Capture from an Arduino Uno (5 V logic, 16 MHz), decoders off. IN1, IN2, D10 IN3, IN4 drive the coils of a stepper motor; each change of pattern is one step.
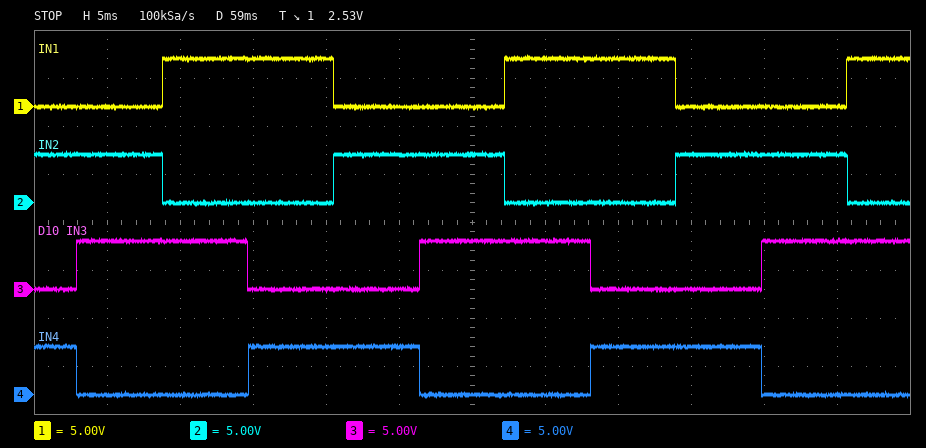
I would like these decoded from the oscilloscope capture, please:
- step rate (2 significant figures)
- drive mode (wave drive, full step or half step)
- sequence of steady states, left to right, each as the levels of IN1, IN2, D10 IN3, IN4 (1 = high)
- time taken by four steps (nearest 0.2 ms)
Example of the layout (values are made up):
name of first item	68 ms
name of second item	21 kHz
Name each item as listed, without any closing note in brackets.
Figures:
step rate	170 steps/s
drive mode	full step
sequence of steady states, left to right, each as the levels of IN1, IN2, D10 IN3, IN4	0101 0110 1010 1001 0101 0110 1010 1001 0101 0110 1010
time taken by four steps	23.4 ms
